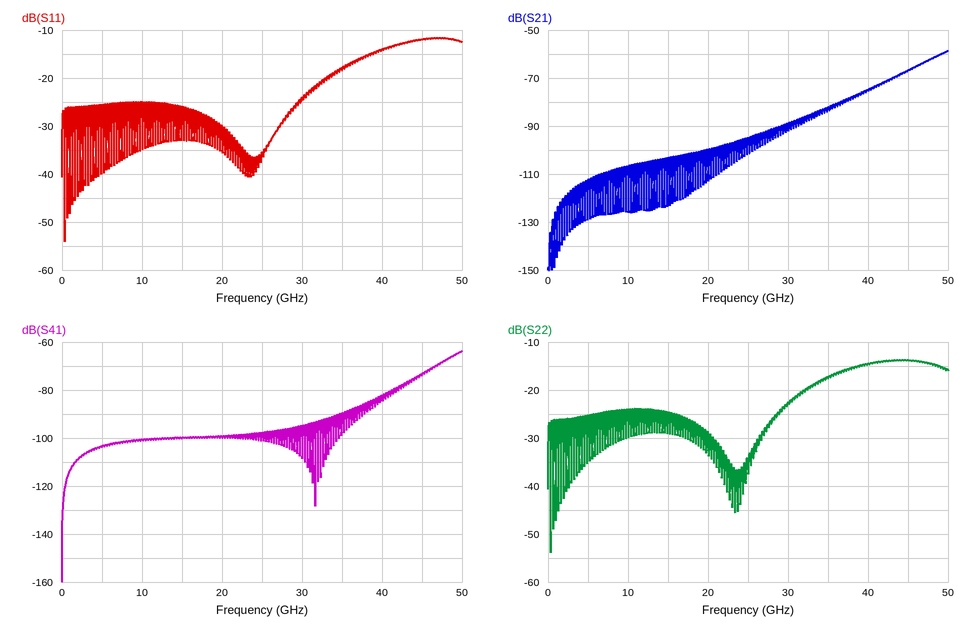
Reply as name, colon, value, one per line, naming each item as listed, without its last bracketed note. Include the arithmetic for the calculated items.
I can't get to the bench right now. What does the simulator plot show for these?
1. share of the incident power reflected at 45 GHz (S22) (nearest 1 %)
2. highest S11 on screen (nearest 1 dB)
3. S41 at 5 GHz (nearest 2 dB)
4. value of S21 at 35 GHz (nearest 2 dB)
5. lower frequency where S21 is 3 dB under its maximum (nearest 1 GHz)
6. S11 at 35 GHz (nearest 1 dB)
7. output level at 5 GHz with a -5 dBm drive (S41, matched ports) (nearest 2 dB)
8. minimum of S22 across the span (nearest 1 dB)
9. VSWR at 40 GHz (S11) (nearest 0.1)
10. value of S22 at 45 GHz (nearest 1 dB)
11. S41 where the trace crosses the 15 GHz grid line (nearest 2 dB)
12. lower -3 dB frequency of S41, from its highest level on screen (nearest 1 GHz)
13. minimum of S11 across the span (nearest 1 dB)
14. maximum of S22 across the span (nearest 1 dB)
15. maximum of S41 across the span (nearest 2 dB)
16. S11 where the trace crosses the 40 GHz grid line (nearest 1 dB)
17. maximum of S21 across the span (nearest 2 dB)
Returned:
share of the incident power reflected at 45 GHz (S22): 10^(-14/10) ≈ 4 %
highest S11 on screen: -12 dB
S41 at 5 GHz: -104 dB
value of S21 at 35 GHz: -82 dB
lower frequency where S21 is 3 dB under its maximum: 48 GHz
S11 at 35 GHz: -18 dB
output level at 5 GHz with a -5 dBm drive (S41, matched ports): -5 dBm + (-104 dB) = -108 dBm
minimum of S22 across the span: -54 dB
VSWR at 40 GHz (S11): |Γ| = 10^(-14/20) = 0.1995; VSWR = (1 + 0.1995)/(1 − 0.1995) ≈ 1.5
value of S22 at 45 GHz: -14 dB
S41 where the trace crosses the 15 GHz grid line: -100 dB
lower -3 dB frequency of S41, from its highest level on screen: 48 GHz
minimum of S11 across the span: -54 dB
maximum of S22 across the span: -14 dB
maximum of S41 across the span: -64 dB
S11 where the trace crosses the 40 GHz grid line: -14 dB
maximum of S21 across the span: -58 dB
